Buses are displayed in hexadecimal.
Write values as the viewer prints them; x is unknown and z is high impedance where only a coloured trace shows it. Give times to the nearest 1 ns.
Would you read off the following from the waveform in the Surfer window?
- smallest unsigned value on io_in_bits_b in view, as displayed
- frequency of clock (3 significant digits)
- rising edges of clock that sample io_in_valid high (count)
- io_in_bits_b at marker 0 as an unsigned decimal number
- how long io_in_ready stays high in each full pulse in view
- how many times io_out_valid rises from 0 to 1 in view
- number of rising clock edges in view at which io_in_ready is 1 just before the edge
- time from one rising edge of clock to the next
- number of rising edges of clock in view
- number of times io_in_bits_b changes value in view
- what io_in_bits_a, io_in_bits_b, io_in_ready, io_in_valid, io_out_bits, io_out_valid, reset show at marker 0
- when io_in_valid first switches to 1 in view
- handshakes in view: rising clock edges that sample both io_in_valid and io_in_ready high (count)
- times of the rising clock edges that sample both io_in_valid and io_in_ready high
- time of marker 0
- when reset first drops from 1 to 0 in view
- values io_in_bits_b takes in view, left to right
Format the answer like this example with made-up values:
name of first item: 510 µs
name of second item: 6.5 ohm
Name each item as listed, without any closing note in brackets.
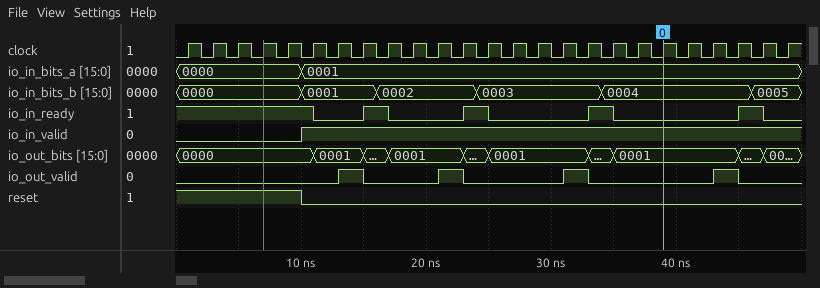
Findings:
smallest unsigned value on io_in_bits_b in view, as displayed: 0000
frequency of clock: 500 MHz
rising edges of clock that sample io_in_valid high: 20
io_in_bits_b at marker 0 as an unsigned decimal number: 4
how long io_in_ready stays high in each full pulse in view: 2 ns, 2 ns, 2 ns, 2 ns
how many times io_out_valid rises from 0 to 1 in view: 4
number of rising clock edges in view at which io_in_ready is 1 just before the edge: 10
time from one rising edge of clock to the next: 2 ns
number of rising edges of clock in view: 25
number of times io_in_bits_b changes value in view: 5
what io_in_bits_a, io_in_bits_b, io_in_ready, io_in_valid, io_out_bits, io_out_valid, reset show at marker 0: io_in_bits_a=0001, io_in_bits_b=0004, io_in_ready=0, io_in_valid=1, io_out_bits=0001, io_out_valid=0, reset=0
when io_in_valid first switches to 1 in view: 10 ns
handshakes in view: rising clock edges that sample both io_in_valid and io_in_ready high: 5
times of the rising clock edges that sample both io_in_valid and io_in_ready high: 11 ns, 17 ns, 25 ns, 35 ns, 47 ns
time of marker 0: 39 ns
when reset first drops from 1 to 0 in view: 10 ns
values io_in_bits_b takes in view, left to right: 0000, 0001, 0002, 0003, 0004, 0005
